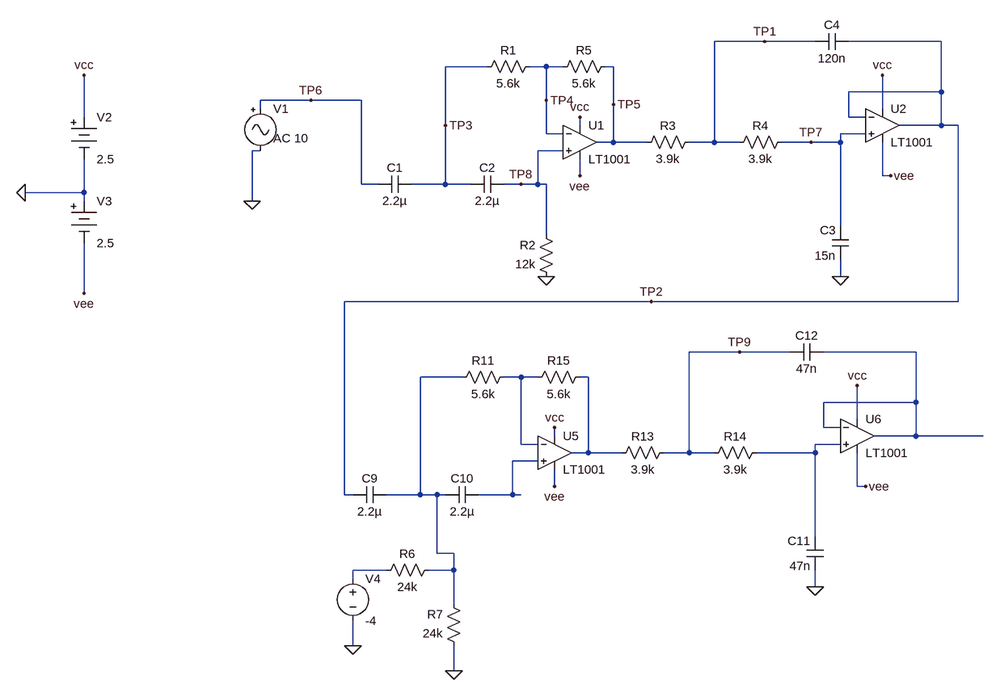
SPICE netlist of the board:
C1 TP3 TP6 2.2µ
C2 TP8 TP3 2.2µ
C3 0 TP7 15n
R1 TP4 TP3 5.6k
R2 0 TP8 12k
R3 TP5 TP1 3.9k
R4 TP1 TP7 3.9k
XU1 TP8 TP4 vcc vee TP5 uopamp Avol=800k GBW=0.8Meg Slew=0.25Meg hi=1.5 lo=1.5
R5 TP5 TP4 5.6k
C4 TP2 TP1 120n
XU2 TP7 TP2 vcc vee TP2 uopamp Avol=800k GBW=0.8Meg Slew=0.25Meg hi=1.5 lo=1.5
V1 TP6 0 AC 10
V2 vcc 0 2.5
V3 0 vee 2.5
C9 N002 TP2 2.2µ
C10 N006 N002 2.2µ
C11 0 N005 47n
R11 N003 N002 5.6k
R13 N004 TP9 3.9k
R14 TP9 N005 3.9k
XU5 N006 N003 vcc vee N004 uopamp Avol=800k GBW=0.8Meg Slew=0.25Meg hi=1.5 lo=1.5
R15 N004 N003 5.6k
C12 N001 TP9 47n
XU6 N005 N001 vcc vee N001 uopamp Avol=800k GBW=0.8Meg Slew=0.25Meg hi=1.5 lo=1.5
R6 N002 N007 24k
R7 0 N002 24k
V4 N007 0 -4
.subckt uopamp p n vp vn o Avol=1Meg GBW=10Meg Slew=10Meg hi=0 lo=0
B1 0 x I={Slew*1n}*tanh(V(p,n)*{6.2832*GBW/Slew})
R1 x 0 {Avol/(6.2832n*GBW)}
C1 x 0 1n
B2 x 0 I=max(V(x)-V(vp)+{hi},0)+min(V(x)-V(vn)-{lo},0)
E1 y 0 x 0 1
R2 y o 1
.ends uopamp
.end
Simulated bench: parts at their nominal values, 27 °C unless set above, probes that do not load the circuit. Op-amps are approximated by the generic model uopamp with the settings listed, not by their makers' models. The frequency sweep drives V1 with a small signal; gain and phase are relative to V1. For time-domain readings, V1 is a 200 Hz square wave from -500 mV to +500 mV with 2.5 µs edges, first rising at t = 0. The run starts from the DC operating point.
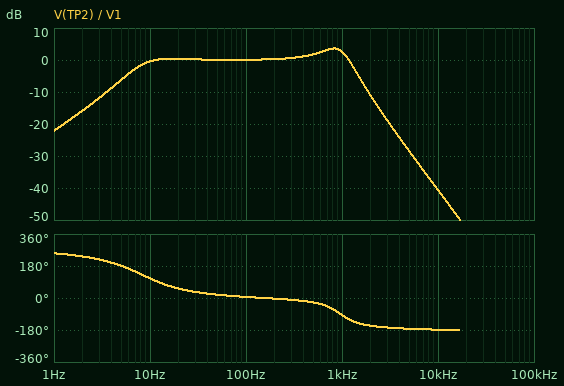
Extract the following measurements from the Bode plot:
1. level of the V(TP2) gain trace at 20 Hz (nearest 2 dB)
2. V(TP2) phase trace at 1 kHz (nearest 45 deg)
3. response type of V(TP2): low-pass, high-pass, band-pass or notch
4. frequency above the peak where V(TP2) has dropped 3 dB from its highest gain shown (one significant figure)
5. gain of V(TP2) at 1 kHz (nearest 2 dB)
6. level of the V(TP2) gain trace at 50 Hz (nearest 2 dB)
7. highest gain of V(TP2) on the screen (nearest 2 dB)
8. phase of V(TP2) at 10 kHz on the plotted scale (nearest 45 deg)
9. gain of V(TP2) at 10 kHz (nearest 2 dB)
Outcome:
0 dB
-90 deg
band-pass
1 kHz
2 dB
0 dB
4 dB
-180 deg
-40 dB
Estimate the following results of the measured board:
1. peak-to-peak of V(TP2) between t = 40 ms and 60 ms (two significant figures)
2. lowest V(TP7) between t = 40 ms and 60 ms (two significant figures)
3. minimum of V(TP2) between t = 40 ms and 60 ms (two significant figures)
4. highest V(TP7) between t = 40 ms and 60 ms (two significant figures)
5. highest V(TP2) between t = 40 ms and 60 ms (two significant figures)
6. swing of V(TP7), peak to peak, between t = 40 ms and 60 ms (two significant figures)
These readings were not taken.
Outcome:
1.7 V
-850 mV
-850 mV
860 mV
860 mV
1.7 V
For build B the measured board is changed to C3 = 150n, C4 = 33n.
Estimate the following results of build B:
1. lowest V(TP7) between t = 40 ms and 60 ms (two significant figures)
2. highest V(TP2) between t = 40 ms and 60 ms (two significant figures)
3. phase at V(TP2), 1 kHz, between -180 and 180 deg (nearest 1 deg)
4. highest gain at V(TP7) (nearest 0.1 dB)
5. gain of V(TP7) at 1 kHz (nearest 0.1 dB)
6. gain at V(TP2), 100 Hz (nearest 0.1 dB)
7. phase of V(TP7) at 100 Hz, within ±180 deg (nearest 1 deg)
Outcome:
-380 mV
390 mV
-104 deg
0.3 dB
-17.6 dB
-1.7 dB
-27 deg
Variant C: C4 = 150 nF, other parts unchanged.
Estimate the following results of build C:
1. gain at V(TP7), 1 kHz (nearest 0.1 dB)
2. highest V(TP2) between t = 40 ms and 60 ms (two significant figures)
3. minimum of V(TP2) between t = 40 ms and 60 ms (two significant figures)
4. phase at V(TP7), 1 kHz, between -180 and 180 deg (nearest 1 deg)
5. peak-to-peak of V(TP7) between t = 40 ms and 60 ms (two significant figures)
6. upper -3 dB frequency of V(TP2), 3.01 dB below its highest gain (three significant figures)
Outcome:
1.8 dB
900 mV
-890 mV
-115 deg
1.8 V
1.02 kHz
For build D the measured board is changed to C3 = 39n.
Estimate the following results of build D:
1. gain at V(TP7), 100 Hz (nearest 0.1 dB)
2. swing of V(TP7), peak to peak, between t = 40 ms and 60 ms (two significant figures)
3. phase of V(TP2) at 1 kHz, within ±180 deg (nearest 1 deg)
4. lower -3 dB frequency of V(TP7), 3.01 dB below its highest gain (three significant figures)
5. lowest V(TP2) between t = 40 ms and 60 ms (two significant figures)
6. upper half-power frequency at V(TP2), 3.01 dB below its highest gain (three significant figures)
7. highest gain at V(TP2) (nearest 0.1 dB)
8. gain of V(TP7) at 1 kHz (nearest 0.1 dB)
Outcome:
0.1 dB
1.3 V
-133 deg
7.29 Hz
-640 mV
676 Hz
0.6 dB
-8.4 dB
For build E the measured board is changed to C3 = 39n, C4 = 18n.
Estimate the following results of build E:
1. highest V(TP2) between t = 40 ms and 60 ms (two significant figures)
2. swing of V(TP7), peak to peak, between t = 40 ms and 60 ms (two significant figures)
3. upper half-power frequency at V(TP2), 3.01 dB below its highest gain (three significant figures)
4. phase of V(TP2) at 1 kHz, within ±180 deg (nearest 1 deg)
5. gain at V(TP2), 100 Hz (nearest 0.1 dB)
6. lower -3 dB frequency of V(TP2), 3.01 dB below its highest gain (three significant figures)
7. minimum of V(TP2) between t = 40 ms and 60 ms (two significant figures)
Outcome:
510 mV
1.0 V
543 Hz
-72 deg
-0.1 dB
7.11 Hz
-500 mV
